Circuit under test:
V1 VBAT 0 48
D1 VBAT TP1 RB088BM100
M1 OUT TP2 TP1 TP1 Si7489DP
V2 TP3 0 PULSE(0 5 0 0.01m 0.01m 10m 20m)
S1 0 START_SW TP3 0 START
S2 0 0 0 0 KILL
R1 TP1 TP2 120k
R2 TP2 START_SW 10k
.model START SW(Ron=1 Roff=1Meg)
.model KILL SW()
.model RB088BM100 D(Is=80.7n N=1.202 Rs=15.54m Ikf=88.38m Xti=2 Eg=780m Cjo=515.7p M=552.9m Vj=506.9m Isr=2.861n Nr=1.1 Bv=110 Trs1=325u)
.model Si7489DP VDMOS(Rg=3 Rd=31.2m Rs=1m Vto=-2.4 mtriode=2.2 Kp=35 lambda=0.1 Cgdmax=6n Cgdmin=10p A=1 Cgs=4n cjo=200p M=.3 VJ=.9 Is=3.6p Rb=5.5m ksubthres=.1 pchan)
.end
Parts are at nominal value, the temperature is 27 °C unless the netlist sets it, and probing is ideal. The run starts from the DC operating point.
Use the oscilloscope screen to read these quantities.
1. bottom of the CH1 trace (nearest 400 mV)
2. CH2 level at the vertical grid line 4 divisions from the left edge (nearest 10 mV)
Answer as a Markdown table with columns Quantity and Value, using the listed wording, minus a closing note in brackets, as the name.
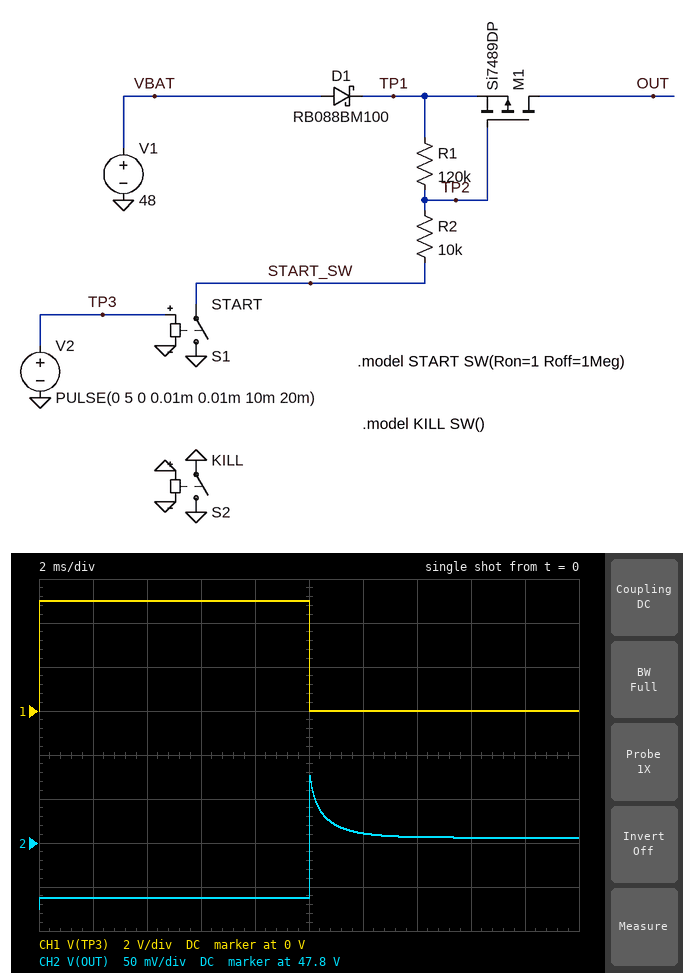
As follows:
| Quantity | Value |
|---|---|
| bottom of the CH1 trace | 0 V |
| CH2 level at the vertical grid line 4 divisions from the left edge | 47.74 V |
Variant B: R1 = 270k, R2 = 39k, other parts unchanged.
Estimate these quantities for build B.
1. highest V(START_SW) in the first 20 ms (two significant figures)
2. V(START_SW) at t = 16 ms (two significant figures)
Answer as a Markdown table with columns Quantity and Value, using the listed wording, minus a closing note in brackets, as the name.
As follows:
| Quantity | Value |
|---|---|
| highest V(START_SW) in the first 20 ms | 36 V |
| V(START_SW) at t = 16 ms | 35 V |
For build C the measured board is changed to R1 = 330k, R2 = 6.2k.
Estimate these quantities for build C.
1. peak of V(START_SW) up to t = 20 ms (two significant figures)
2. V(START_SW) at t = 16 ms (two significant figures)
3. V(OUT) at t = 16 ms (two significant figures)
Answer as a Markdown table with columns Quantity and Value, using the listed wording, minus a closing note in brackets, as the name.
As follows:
| Quantity | Value |
|---|---|
| peak of V(START_SW) up to t = 20 ms | 35 V |
| V(START_SW) at t = 16 ms | 33 V |
| V(OUT) at t = 16 ms | 48 V |
